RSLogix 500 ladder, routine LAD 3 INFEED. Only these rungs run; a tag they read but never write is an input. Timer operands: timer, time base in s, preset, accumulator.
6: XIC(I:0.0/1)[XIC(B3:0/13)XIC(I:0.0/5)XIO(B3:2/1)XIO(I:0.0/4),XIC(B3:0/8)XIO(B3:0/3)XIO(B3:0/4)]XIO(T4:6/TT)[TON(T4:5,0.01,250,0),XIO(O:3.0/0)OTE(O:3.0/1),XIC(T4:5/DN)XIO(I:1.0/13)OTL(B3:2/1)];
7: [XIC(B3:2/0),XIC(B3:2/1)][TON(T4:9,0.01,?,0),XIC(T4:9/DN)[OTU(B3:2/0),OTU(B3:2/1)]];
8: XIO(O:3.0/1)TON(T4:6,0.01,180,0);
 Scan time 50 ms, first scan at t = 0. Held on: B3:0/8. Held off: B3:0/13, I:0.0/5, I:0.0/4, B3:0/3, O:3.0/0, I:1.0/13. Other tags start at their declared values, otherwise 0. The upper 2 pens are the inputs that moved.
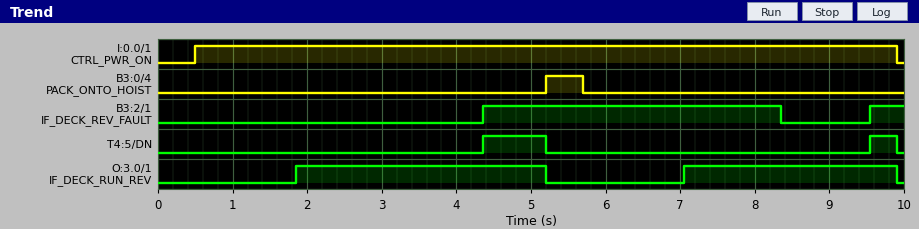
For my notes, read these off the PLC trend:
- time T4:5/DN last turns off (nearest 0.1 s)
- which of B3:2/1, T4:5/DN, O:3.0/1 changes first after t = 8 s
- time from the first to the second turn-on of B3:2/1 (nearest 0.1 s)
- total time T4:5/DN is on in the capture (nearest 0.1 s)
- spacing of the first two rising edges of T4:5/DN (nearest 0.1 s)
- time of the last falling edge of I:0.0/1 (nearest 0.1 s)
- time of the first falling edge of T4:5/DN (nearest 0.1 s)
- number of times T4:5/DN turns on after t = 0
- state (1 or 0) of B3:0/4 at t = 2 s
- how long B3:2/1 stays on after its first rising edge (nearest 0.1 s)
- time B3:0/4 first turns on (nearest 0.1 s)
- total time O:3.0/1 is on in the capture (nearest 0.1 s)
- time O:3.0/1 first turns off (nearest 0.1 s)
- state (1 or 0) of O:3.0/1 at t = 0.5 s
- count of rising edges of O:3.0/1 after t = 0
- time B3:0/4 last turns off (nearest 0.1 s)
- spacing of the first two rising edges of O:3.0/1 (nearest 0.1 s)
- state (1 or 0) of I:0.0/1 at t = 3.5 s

9.9 s
B3:2/1
5.2 s
1.2 s
5.2 s
9.9 s
5.2 s
2
0
4.0 s
5.2 s
6.2 s
5.2 s
0
2
5.7 s
5.2 s
1
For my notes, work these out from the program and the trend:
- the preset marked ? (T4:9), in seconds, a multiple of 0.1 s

4.0 s
